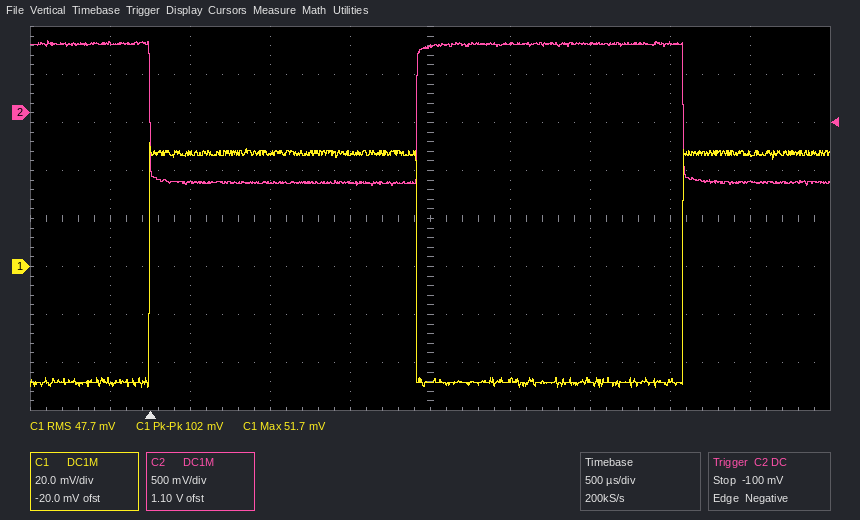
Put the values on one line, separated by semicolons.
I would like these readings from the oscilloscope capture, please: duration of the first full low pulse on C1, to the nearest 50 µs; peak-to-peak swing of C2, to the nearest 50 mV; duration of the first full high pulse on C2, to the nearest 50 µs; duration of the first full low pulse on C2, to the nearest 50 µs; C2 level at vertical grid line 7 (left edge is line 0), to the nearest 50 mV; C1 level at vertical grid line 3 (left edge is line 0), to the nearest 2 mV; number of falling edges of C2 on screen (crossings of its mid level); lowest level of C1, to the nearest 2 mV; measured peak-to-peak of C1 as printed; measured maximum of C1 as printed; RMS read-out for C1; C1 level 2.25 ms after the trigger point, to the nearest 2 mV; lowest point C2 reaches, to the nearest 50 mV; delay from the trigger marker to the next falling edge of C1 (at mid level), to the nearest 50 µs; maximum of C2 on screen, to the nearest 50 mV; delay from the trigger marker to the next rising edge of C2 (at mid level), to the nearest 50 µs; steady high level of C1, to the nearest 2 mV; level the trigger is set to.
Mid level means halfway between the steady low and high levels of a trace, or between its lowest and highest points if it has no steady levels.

1.65 ms; 1.50 V; 1.65 ms; 1.65 ms; 700 mV; 48 mV; 2; -50 mV; 102 mV; 51.7 mV; 47.7 mV; -48 mV; -750 mV; 1.65 ms; 750 mV; 1.65 ms; 48 mV; -100 mV
